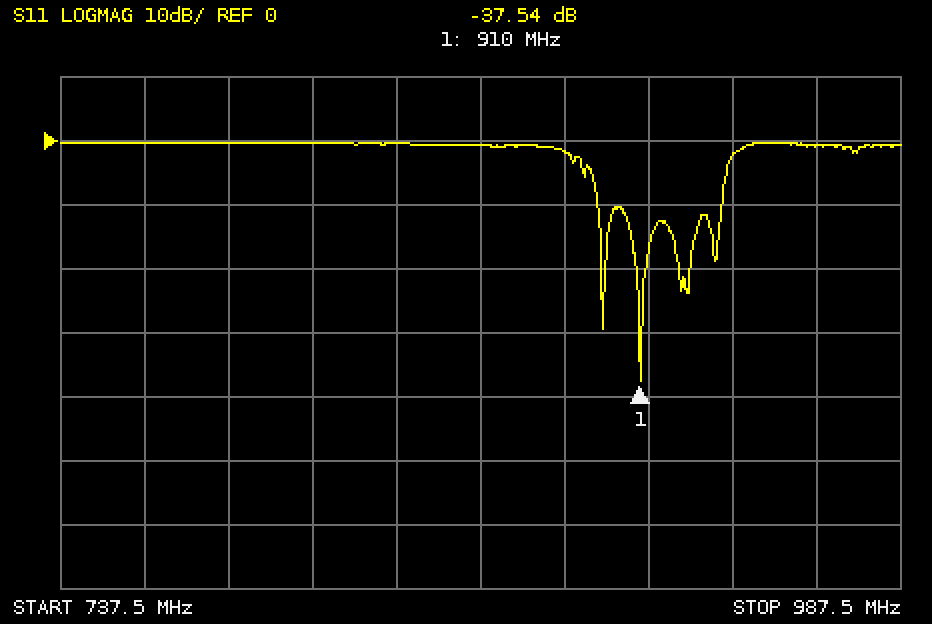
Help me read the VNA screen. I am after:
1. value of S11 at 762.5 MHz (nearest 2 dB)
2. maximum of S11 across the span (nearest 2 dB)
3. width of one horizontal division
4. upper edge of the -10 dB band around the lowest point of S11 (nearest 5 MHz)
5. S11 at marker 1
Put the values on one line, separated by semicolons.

0 dB; 0 dB; 25 MHz; 935 MHz; -37.54 dB
